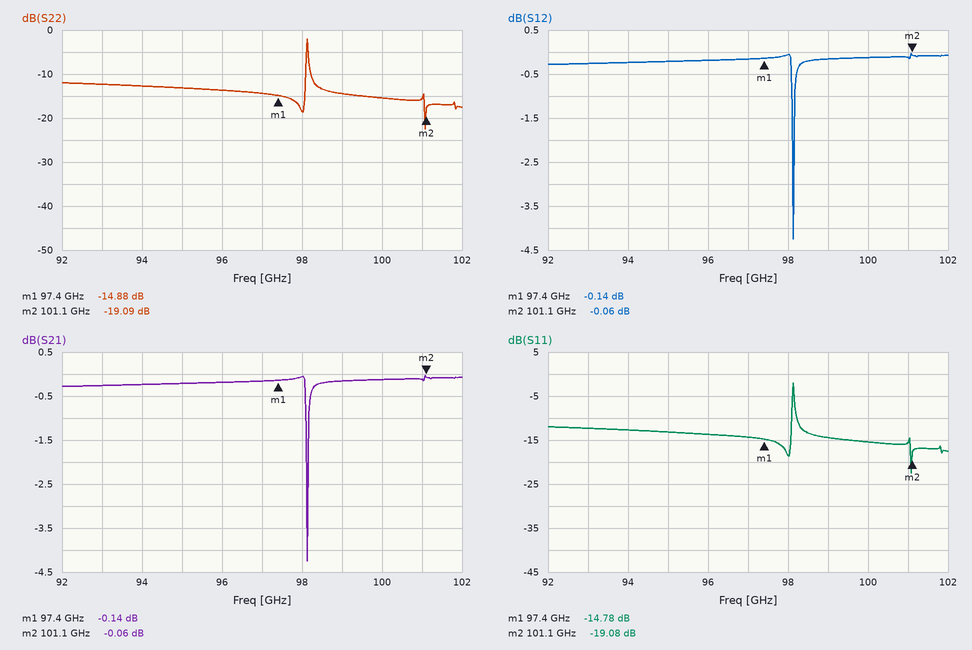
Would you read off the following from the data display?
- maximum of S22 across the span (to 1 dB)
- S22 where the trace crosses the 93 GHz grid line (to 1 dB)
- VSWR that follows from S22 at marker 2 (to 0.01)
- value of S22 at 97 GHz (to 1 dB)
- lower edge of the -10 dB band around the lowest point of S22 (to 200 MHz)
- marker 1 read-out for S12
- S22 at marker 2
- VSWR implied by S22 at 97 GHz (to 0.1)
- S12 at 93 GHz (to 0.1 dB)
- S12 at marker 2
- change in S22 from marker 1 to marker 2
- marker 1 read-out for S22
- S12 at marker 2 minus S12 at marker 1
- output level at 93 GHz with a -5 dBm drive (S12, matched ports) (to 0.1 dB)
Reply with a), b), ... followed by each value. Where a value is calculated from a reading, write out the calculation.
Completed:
a) -2 dB
b) -12 dB
c) (1 + 0.1110)/(1 − 0.1110) ≈ 1.25
d) -14 dB
e) 98.2 GHz
f) -0.14 dB
g) -19.09 dB
h) |Γ| = 10^(-14/20) = 0.1995; VSWR = (1 + 0.1995)/(1 − 0.1995) ≈ 1.5
i) -0.3 dB
j) -0.06 dB
k) -19.09 − (-14.88) = -4.21 dB
l) -14.88 dB
m) -0.06 − (-0.14) = 0.08 dB
n) -5 dBm + (-0.3 dB) = -5.3 dBm
